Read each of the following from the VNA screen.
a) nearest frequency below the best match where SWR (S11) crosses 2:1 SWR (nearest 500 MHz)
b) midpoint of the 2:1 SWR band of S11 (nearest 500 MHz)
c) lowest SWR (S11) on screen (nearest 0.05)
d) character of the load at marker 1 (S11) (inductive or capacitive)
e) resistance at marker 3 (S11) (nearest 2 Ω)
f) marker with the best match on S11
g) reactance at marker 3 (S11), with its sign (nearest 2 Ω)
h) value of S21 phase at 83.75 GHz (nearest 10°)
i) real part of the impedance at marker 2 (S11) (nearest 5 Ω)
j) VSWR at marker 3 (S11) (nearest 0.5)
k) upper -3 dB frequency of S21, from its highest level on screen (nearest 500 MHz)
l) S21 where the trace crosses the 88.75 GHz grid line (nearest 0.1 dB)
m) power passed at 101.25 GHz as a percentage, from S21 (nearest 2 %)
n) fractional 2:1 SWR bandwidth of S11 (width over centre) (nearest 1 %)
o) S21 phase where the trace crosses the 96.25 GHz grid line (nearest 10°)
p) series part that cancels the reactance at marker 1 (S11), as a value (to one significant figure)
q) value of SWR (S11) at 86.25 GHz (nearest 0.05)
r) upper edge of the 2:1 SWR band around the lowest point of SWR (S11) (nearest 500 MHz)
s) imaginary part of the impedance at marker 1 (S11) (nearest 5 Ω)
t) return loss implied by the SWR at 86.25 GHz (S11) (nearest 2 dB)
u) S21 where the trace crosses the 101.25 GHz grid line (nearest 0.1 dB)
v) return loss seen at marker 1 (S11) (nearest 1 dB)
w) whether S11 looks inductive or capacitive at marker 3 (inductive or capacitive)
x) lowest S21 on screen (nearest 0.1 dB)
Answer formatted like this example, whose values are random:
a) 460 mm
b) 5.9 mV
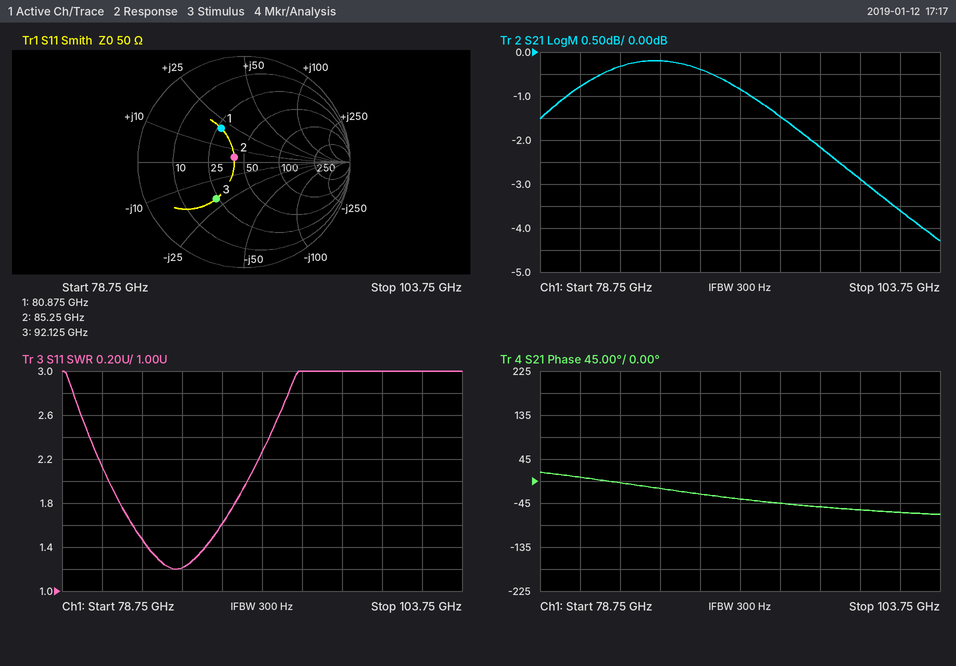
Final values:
a) 81.5 GHz
b) 86.0 GHz
c) 1.20
d) inductive
e) 24 Ω
f) marker 2
g) -20 Ω
h) 0°
i) 40 Ω
j) 2.5
k) 100.0 GHz
l) -0.4 dB
m) 44 %
n) 10 %
o) -50°
p) 100 fF
q) 1.20
r) 90.5 GHz
s) +20 Ω
t) 20 dB
u) -3.6 dB
v) 8 dB
w) capacitive
x) -4.3 dB
